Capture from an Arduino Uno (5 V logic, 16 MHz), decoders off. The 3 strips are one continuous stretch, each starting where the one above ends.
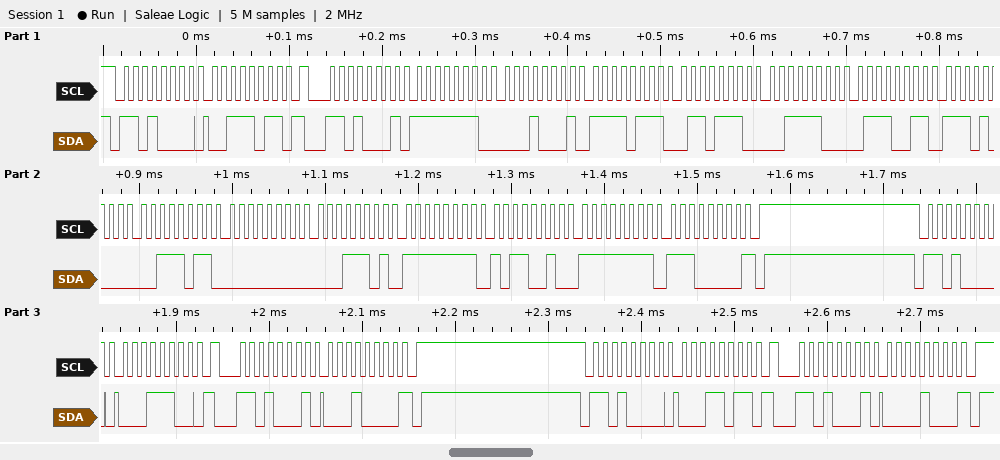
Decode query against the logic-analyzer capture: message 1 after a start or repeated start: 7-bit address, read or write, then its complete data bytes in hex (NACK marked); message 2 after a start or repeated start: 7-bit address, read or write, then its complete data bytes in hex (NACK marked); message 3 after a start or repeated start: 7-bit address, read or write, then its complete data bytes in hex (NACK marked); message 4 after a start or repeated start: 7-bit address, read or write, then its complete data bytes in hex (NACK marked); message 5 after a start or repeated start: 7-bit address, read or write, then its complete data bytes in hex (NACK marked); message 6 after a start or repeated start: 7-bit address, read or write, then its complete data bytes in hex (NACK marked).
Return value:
0x68 write: 3B
0x68 read: FE 11 F7 6E 3C 73 E8 3B 00 1D FF B2 FF E0 NACK
0x68 write: 1C
0x68 read: 10 NACK
0x68 write: 1B
0x68 read: 08 NACK
